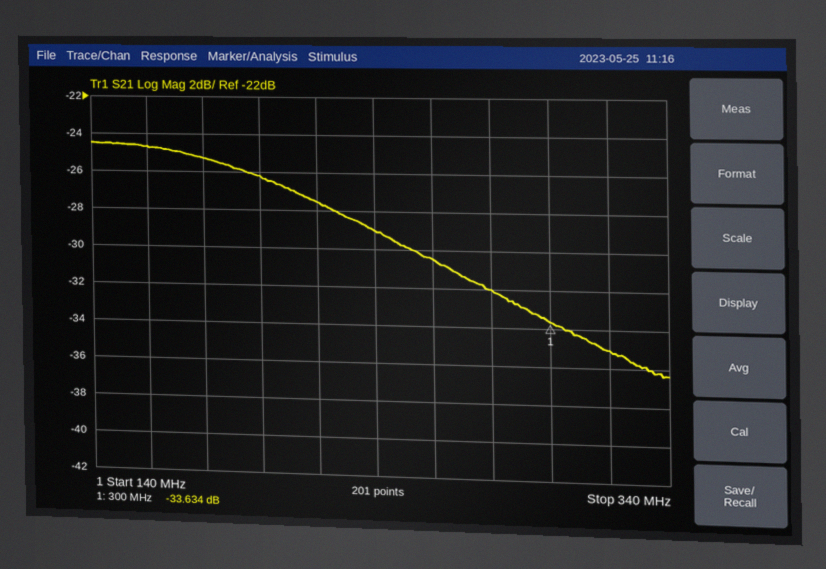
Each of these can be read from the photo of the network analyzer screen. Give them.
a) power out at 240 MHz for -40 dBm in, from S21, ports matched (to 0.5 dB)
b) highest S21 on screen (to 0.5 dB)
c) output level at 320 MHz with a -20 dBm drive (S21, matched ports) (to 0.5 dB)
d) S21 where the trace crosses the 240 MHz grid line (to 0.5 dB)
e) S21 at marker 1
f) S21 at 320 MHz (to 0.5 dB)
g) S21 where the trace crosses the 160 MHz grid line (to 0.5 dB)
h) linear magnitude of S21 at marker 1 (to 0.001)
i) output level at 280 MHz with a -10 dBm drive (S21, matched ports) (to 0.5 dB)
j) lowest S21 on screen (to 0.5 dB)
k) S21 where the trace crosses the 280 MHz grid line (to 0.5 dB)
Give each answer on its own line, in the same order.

-69.0 dBm
-24.5 dB
-55.0 dBm
-29.0 dB
-33.634 dB
-35.0 dB
-24.5 dB
0.021
-42.0 dBm
-36.5 dB
-32.0 dB
